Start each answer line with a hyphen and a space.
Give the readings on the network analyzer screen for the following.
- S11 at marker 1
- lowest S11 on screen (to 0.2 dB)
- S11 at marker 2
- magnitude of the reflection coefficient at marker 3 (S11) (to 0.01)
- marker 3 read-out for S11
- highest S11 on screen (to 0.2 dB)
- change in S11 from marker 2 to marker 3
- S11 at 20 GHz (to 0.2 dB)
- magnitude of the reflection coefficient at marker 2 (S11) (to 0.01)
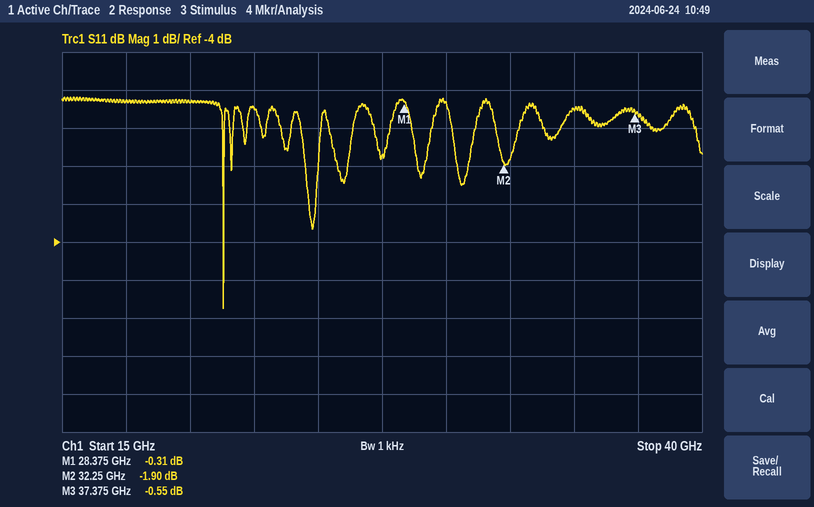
- -0.31 dB
- -5.8 dB
- -1.90 dB
- 0.94
- -0.55 dB
- -0.2 dB
- 1.35 dB
- -0.4 dB
- 0.80
